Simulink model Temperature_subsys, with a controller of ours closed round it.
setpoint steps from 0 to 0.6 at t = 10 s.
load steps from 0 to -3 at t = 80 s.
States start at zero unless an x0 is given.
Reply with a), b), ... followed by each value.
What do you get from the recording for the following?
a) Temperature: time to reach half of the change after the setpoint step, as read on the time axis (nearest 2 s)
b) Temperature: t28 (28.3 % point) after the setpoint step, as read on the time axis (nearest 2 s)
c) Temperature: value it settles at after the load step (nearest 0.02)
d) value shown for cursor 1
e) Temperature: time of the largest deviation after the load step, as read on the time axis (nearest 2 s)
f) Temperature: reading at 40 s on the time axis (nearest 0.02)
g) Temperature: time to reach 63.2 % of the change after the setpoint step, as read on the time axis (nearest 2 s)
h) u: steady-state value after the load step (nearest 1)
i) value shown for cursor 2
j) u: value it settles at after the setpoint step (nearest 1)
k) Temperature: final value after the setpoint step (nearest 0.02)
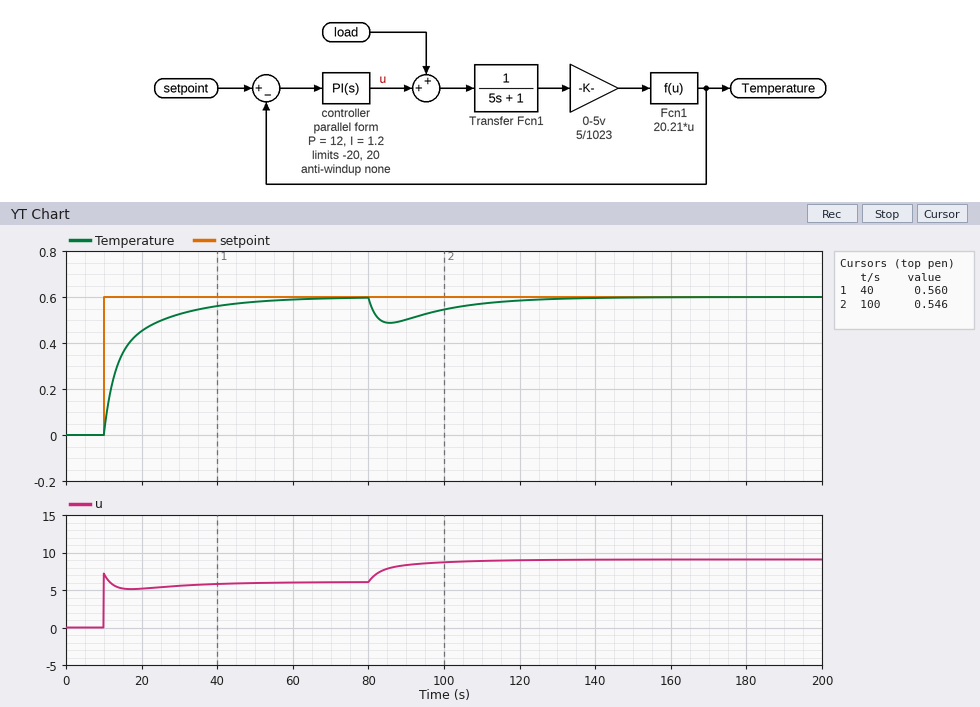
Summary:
a) 14 s
b) 12 s
c) 0.60
d) 0.560
e) 86 s
f) 0.56
g) 16 s
h) 9
i) 0.546
j) 6
k) 0.60
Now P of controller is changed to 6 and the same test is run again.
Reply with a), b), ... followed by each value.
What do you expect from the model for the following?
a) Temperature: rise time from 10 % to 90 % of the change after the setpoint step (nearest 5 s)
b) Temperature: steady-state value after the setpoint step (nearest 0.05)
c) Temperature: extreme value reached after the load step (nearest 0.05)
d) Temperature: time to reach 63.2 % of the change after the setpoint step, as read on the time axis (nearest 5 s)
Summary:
a) 20 s
b) 0.60
c) 0.45
d) 20 s
